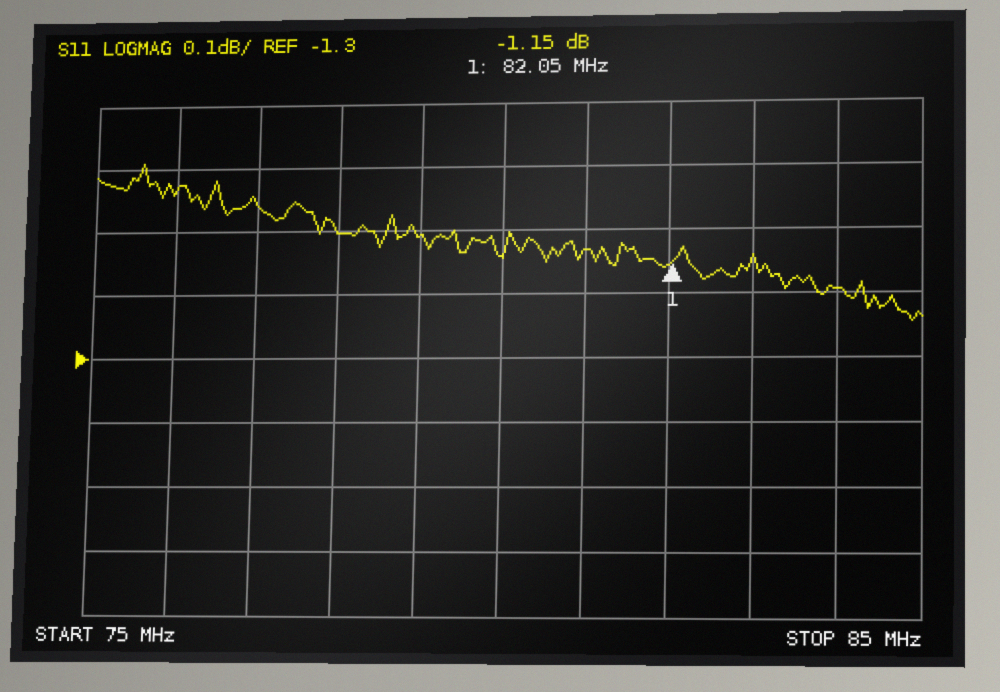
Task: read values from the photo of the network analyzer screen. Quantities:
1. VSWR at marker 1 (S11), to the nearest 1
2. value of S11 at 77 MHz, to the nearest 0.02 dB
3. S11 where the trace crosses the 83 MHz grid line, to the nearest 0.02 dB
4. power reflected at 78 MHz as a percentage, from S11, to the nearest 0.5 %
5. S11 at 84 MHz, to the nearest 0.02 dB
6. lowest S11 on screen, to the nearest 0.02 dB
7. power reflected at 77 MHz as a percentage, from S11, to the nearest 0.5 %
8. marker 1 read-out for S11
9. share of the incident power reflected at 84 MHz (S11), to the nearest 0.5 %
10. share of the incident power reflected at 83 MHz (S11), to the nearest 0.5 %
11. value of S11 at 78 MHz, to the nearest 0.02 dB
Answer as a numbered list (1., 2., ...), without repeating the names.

1. 15
2. -1.06 dB
3. -1.14 dB
4. 77.5 %
5. -1.20 dB
6. -1.24 dB
7. 78.5 %
8. -1.15 dB
9. 76.0 %
10. 77.0 %
11. -1.10 dB
